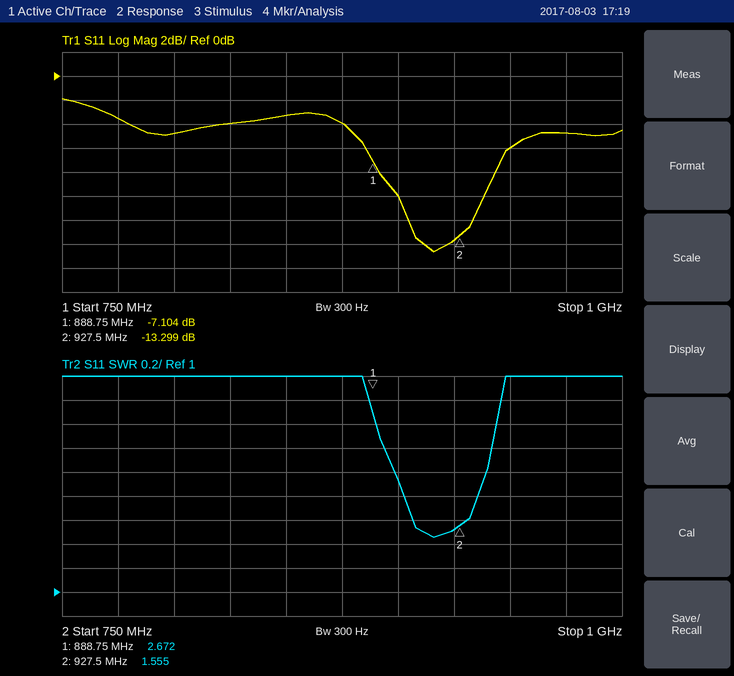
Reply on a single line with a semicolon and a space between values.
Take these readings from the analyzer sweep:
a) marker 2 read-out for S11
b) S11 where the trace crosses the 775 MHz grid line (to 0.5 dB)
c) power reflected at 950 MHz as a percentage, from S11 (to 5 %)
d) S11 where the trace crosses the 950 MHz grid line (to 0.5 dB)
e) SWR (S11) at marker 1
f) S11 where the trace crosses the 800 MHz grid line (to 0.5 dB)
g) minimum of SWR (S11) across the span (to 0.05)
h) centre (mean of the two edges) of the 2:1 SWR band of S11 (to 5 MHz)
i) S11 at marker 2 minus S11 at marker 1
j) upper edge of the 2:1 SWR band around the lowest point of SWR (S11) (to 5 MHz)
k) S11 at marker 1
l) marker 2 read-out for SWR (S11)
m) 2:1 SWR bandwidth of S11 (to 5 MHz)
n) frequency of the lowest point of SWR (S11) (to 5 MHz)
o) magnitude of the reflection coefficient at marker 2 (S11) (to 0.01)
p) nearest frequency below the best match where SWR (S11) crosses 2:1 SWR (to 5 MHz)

-13.299 dB; -3.5 dB; 25 %; -6.0 dB; 2.672; -5.0 dB; 1.45; 920 MHz; -6.195 dB; 940 MHz; -7.104 dB; 1.555; 40 MHz; 915 MHz; 0.22; 900 MHz
